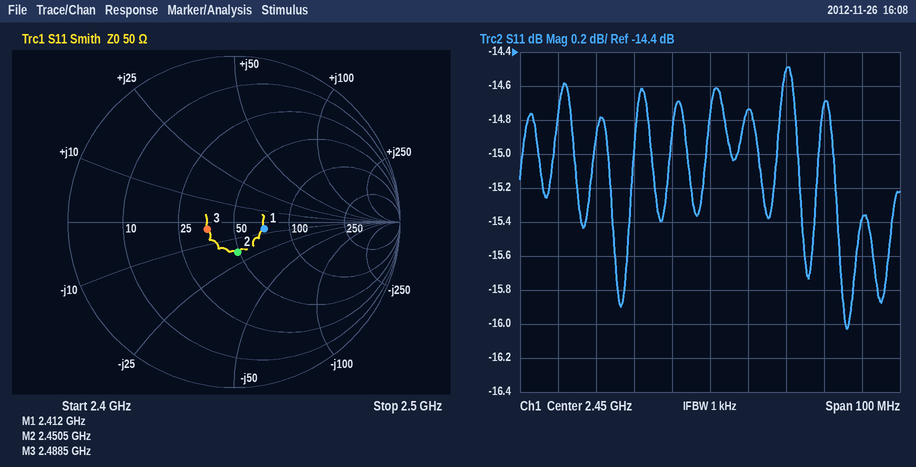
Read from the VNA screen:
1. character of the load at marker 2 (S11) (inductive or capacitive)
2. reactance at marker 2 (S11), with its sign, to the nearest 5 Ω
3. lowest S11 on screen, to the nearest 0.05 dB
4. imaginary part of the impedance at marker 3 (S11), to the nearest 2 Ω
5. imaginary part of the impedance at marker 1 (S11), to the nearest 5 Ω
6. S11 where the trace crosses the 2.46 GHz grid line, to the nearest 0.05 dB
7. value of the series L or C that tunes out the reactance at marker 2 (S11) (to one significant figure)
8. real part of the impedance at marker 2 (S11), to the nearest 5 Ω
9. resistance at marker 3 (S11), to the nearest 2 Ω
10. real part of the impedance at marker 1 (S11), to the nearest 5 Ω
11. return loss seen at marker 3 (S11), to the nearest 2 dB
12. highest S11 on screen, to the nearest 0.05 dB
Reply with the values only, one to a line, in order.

capacitive
-20 Ω
-16.05 dB
-4 Ω
-5 Ω
-14.75 dB
1 nH
50 Ω
36 Ω
70 Ω
16 dB
-14.50 dB
